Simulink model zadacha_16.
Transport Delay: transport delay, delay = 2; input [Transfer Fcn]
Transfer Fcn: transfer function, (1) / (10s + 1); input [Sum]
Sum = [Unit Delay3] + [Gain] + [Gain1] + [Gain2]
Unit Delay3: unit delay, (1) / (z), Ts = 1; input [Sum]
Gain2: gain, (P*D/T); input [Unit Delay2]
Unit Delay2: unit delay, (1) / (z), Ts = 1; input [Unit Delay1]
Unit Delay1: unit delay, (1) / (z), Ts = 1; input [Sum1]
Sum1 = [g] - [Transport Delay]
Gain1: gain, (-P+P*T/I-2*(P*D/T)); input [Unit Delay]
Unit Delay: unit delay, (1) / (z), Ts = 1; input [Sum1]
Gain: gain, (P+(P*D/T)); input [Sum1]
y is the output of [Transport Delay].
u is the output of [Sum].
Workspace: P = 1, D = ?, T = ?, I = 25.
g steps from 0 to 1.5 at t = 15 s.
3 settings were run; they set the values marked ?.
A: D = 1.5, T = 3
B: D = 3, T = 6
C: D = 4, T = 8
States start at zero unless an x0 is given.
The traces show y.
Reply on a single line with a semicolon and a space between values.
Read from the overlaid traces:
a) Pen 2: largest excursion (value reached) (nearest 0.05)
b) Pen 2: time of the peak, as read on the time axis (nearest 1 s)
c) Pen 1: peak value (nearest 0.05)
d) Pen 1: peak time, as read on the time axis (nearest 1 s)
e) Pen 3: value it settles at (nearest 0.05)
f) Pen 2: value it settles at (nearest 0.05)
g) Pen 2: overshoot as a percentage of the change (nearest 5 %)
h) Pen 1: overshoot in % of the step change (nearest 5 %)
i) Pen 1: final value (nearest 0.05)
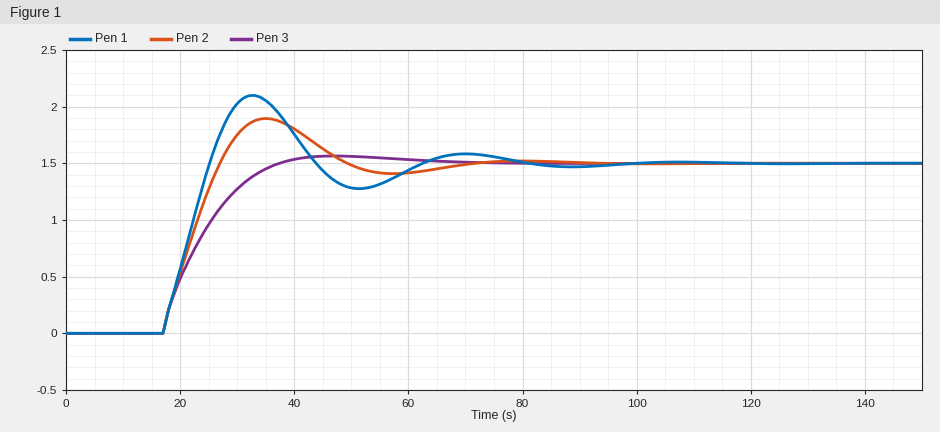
1.90; 35 s; 2.10; 33 s; 1.50; 1.50; 25 %; 40 %; 1.50
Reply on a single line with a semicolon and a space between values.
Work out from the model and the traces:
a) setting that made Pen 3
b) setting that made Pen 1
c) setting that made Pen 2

A; C; B
